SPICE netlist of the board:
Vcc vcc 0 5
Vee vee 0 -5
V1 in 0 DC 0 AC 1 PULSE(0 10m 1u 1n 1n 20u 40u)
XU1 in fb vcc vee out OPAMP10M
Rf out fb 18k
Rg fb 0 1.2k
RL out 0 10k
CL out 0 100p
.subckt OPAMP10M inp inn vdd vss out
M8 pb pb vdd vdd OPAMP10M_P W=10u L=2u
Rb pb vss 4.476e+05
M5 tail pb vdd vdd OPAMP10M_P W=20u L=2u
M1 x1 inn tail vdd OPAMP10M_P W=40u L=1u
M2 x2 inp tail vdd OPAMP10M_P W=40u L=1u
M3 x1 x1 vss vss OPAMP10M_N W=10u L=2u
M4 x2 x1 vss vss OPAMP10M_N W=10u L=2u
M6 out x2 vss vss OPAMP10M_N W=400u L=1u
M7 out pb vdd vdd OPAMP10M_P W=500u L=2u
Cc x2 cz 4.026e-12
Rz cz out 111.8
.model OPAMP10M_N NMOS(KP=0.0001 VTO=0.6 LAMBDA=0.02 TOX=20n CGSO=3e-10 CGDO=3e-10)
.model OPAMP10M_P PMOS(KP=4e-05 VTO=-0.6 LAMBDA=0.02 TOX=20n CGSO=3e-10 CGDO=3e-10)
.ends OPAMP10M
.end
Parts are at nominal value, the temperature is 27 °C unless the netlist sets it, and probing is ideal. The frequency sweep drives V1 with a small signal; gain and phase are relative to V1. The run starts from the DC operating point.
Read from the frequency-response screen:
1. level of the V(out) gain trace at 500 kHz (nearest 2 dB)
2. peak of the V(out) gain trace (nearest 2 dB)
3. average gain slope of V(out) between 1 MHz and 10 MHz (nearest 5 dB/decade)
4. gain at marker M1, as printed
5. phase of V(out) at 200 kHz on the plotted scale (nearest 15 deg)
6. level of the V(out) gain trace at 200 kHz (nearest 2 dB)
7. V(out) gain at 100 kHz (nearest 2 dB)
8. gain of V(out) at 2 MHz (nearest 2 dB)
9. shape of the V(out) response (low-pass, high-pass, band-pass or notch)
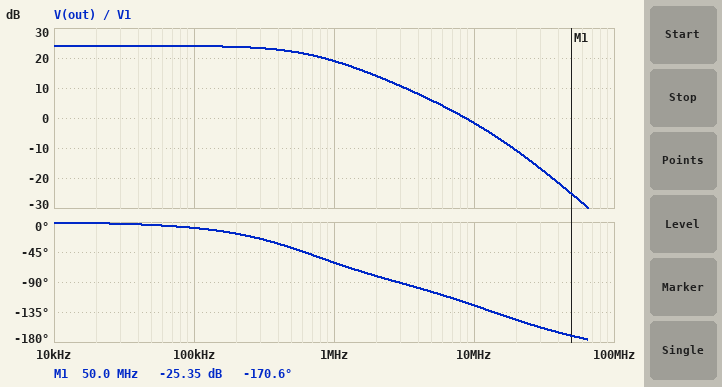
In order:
22 dB
24 dB
-20 dB/decade
-25.35 dB
-15 deg
24 dB
24 dB
14 dB
low-pass
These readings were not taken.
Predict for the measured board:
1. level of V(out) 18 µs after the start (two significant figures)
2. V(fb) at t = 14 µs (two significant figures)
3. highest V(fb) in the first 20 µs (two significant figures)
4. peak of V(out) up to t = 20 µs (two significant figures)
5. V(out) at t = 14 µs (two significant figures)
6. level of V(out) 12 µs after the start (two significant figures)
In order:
160 mV
9.8 mV
9.8 mV
160 mV
160 mV
160 mV
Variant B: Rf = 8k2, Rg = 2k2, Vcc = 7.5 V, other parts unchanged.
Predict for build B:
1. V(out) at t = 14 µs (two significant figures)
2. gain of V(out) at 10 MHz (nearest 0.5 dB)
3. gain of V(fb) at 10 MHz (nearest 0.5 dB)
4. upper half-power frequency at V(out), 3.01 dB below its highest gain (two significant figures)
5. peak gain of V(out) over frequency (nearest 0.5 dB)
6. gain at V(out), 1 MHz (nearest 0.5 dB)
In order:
46 mV
0.5 dB
-13.0 dB
3.0 MHz
13.5 dB
13.0 dB
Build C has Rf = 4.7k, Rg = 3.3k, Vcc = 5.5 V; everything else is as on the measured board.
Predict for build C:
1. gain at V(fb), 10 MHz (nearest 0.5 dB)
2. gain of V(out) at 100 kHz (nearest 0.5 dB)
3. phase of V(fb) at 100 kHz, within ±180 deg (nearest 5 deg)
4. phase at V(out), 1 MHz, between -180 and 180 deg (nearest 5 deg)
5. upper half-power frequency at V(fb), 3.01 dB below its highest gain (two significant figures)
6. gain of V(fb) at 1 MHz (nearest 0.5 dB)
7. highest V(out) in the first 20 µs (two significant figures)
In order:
-8.0 dB
7.5 dB
0 deg
-15 deg
5.8 MHz
0 dB
24 mV
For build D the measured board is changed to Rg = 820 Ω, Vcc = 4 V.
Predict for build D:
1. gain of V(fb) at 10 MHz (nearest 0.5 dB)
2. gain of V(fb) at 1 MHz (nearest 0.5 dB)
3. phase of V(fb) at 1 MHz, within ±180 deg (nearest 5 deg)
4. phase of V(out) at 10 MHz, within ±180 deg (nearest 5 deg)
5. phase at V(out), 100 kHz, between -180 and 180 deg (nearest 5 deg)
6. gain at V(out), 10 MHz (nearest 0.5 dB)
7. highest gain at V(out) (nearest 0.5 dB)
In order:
-30.0 dB
-8.0 dB
-70 deg
-130 deg
-15 deg
-2.5 dB
27.0 dB
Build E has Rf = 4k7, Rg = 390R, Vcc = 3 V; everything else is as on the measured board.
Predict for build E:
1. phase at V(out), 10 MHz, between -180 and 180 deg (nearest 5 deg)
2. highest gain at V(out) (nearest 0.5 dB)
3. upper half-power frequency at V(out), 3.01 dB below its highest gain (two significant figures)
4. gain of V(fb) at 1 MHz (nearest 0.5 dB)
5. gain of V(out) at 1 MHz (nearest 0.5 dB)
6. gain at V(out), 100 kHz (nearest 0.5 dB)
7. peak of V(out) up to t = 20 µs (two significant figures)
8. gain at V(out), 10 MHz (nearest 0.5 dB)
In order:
-130 deg
22.5 dB
710 kHz
-5.0 dB
17.5 dB
22.0 dB
130 mV
-3.5 dB
